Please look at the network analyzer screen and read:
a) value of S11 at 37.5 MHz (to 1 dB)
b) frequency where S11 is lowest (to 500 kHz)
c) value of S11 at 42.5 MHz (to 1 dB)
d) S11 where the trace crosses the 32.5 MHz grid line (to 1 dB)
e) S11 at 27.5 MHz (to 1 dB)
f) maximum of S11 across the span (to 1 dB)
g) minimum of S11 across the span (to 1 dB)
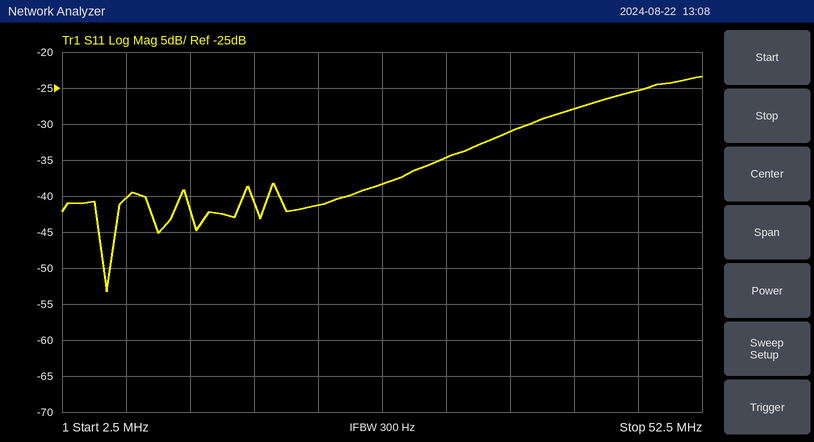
-31 dB
6.0 MHz
-28 dB
-35 dB
-38 dB
-23 dB
-53 dB
